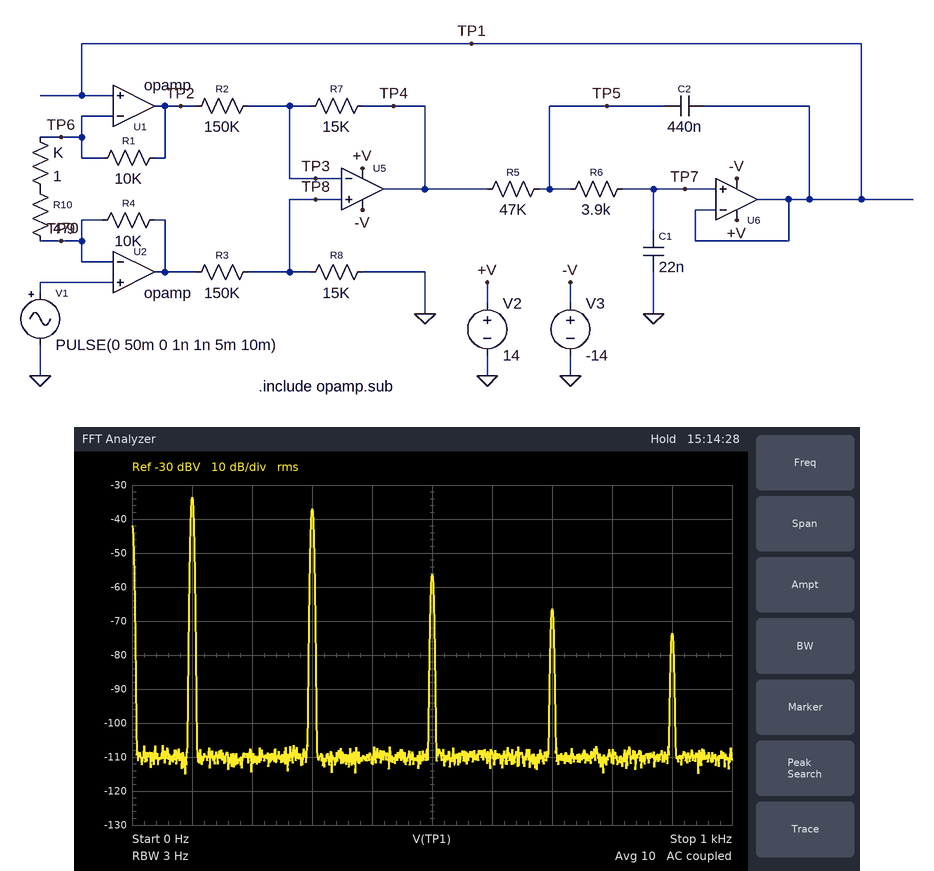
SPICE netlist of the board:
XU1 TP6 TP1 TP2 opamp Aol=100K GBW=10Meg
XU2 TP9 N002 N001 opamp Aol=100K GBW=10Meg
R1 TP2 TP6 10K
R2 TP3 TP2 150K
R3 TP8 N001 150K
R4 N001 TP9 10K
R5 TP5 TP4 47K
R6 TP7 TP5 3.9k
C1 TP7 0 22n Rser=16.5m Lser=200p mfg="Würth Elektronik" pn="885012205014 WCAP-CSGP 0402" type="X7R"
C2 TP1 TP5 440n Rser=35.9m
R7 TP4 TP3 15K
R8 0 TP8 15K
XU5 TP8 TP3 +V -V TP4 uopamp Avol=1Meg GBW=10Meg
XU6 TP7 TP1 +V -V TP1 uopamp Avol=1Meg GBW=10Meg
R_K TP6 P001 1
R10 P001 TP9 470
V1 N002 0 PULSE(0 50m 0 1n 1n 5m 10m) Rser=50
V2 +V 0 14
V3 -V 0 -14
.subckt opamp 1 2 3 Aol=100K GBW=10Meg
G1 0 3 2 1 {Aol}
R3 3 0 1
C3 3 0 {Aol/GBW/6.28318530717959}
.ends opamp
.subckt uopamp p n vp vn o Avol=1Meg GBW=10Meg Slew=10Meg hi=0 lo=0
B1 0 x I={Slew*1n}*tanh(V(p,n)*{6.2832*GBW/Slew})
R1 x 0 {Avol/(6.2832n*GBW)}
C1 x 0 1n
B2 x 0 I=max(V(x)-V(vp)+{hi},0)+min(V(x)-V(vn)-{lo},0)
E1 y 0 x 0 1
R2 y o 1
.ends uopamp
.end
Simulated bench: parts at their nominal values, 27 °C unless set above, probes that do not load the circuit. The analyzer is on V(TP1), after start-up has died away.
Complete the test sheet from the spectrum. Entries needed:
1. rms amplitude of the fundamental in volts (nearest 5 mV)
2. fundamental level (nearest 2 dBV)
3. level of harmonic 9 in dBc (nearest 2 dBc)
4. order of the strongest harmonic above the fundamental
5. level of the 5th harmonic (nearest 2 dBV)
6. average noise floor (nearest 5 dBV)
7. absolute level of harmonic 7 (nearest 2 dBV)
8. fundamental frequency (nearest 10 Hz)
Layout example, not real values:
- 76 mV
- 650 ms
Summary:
- 20 mV
- -34 dBV
- -40 dBc
- 3
- -56 dBV
- -110 dBV
- -66 dBV
- 100 Hz
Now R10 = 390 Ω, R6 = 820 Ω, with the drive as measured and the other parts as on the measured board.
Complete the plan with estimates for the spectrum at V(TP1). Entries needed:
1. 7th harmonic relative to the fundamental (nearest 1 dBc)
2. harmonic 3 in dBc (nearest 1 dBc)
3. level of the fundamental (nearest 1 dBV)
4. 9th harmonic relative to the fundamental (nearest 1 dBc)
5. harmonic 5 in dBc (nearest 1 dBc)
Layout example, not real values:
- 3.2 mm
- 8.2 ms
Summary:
- -15 dBc
- -8 dBc
- -34 dBV
- -22 dBc
- -11 dBc
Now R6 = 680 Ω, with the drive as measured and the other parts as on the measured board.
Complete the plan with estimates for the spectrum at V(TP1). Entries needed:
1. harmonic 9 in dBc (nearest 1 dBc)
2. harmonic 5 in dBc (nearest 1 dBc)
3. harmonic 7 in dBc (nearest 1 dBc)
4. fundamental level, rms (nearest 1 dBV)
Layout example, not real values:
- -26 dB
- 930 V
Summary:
- -22 dBc
- -12 dBc
- -16 dBc
- -35 dBV
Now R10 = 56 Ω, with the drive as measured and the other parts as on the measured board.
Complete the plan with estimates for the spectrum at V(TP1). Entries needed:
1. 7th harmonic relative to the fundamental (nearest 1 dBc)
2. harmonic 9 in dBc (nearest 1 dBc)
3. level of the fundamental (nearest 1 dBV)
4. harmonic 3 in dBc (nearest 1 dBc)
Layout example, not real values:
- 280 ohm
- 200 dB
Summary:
- 1 dBc
- -15 dBc
- -33 dBV
- -8 dBc
